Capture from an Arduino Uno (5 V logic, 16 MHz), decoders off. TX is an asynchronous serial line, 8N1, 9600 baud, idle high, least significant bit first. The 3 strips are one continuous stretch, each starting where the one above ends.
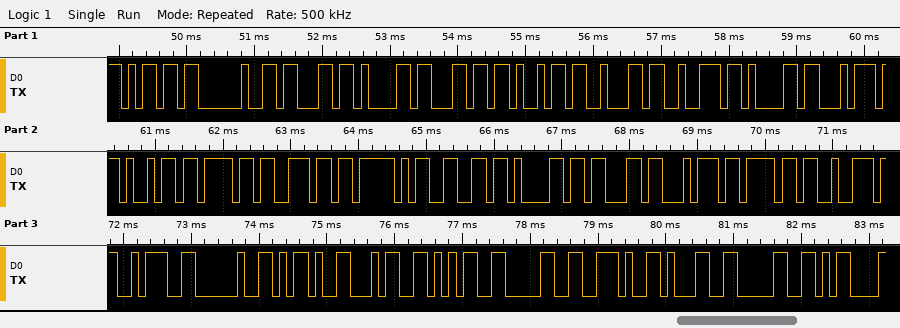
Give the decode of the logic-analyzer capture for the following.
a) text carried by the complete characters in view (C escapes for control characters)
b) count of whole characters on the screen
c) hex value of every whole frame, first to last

"m calibration_factor: -450.10\r"
30
6D 20 63 61 6C 69 62 72 61 74 69 6F 6E 5F 66 61 63 74 6F 72 3A 20 2D 34 35 30 2E 31 30 0D
